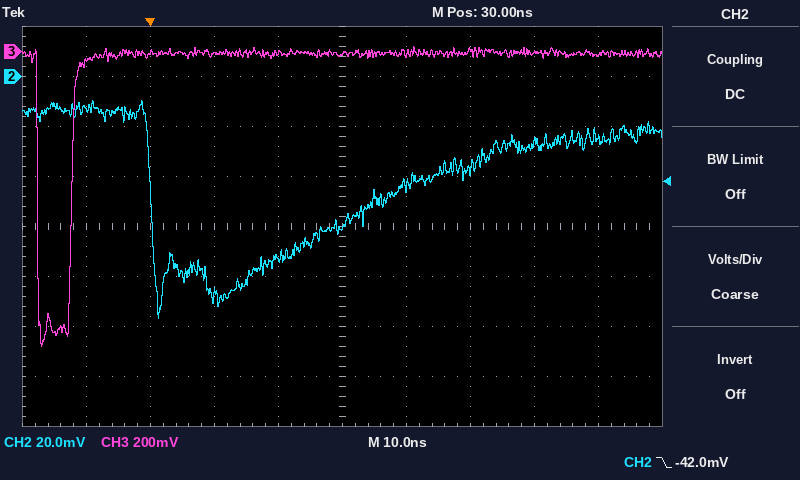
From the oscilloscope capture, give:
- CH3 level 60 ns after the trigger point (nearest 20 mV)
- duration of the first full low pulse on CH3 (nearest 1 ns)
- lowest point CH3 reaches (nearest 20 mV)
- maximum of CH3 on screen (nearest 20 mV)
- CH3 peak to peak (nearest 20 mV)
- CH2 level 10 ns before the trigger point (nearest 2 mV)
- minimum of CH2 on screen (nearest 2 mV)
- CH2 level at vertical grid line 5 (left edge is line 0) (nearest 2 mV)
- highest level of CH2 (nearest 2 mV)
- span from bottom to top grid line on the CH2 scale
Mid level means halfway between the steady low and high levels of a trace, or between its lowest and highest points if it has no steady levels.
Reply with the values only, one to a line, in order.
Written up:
0 mV
5 ns
-1.18 V
20 mV
1.20 V
-12 mV
-96 mV
-60 mV
-10 mV
160 mV
